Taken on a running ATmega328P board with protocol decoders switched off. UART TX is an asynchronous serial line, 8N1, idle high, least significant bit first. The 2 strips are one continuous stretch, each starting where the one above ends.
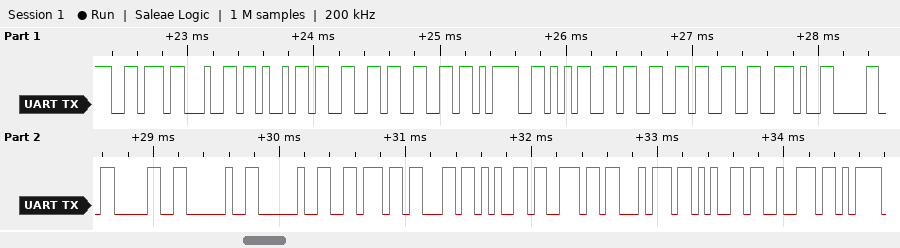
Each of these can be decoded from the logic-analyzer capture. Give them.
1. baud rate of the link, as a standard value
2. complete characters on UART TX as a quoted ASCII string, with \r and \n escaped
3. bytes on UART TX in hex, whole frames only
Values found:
19200 baud
"vdiff=533.00  vcenter"
0x76 0x64 0x69 0x66 0x66 0x3D 0x35 0x33 0x33 0x2E 0x30 0x30 0x20 0x20 0x76 0x63 0x65 0x6E 0x74 0x65 0x72
